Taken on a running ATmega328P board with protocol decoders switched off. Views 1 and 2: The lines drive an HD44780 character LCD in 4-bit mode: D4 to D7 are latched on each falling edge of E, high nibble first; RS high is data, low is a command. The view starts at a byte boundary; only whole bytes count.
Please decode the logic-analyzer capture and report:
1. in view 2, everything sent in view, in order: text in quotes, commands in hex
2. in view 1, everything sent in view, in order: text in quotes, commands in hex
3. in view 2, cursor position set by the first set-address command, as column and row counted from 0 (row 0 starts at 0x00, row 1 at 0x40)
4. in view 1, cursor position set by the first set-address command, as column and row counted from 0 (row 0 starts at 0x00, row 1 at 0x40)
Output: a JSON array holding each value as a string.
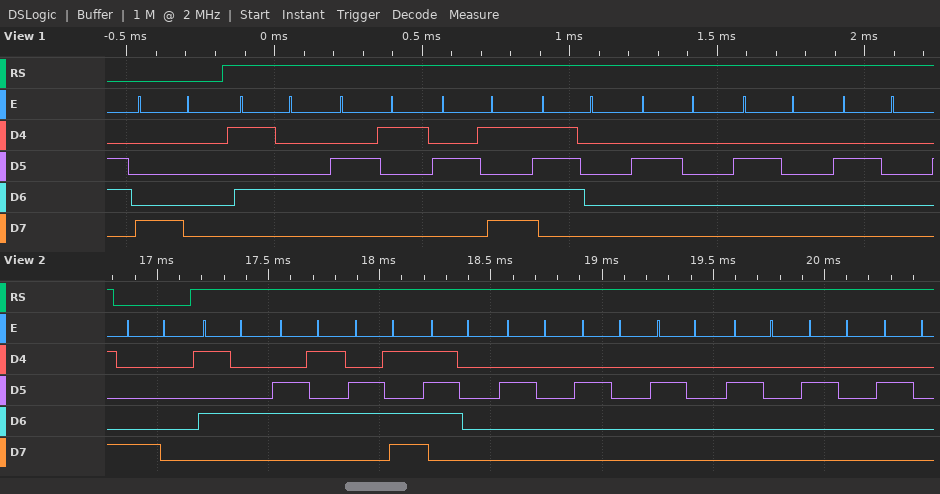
["0x80 \"Temp      \"", "0x80 \"Temp   \"", "column 0, row 0", "column 0, row 0"]
